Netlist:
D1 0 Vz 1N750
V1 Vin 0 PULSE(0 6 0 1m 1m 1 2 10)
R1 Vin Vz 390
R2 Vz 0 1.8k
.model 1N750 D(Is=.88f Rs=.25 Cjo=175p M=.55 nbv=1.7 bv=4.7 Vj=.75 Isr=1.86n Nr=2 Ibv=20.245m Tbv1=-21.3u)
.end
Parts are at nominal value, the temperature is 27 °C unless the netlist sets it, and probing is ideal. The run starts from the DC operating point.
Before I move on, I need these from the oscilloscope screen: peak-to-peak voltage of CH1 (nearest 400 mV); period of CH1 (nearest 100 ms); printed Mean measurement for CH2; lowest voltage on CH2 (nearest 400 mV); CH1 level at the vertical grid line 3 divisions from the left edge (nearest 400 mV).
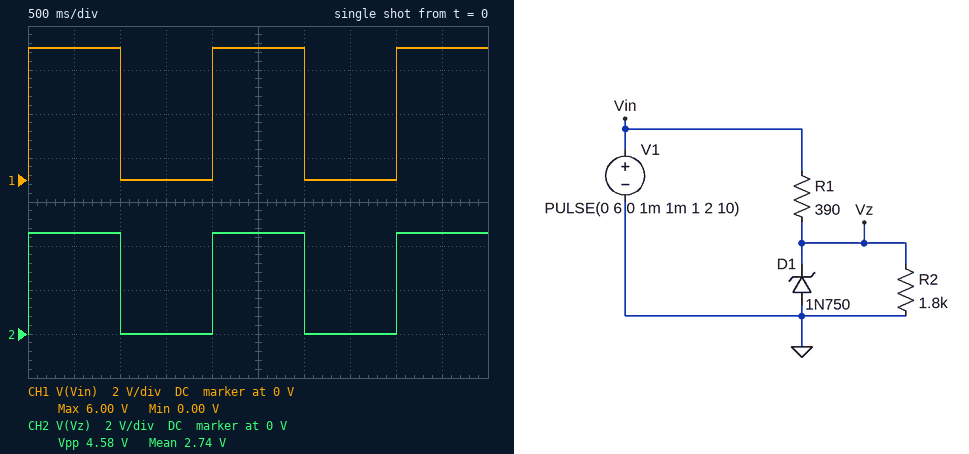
6.0 V
2.0 s
2.74 V
0 V
0 V
